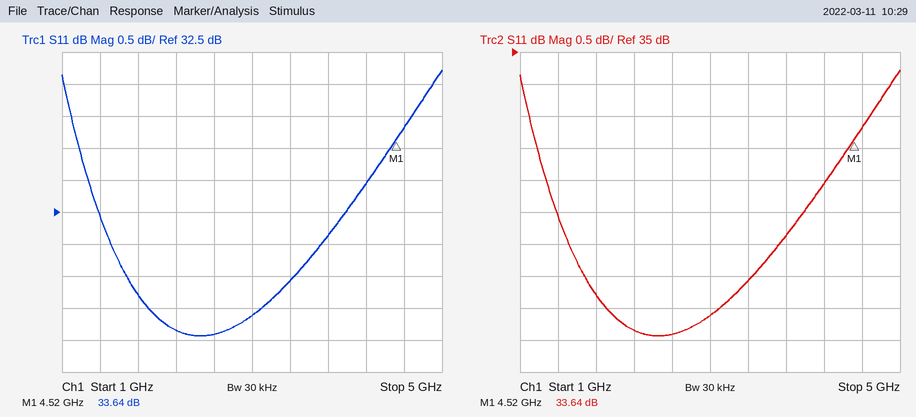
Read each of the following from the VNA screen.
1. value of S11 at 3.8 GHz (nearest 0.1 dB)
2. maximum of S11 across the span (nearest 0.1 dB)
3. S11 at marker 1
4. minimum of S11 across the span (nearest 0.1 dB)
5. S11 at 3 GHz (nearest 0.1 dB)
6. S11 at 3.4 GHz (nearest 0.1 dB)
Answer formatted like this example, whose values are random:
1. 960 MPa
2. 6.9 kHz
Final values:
1. 32.1 dB
2. 34.7 dB
3. 33.64 dB
4. 30.6 dB
5. 30.9 dB
6. 31.4 dB
